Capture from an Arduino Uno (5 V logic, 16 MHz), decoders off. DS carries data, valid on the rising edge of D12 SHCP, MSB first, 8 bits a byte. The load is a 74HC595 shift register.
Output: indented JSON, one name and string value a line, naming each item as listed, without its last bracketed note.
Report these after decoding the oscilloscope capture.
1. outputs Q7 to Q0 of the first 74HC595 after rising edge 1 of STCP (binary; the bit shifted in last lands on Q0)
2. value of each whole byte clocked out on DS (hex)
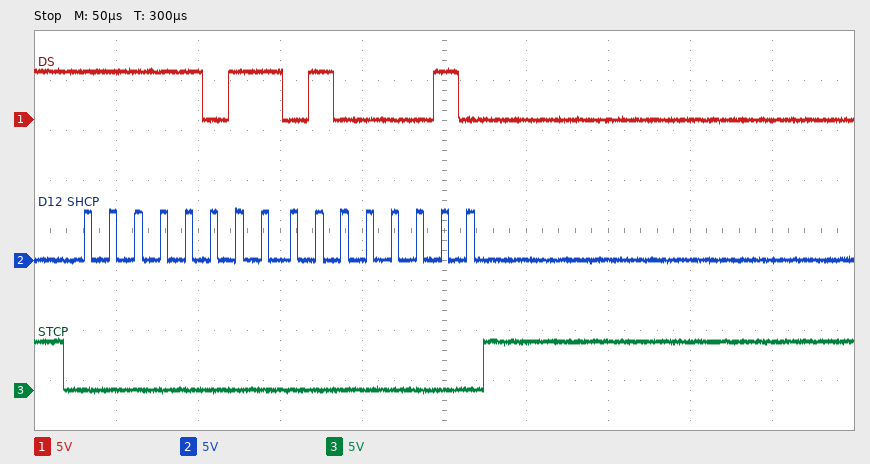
{
  "outputs Q7 to Q0 of the first 74HC595 after rising edge 1 of STCP": "01000010",
  "value of each whole byte clocked out on DS": "0xFB 0x42"
}
